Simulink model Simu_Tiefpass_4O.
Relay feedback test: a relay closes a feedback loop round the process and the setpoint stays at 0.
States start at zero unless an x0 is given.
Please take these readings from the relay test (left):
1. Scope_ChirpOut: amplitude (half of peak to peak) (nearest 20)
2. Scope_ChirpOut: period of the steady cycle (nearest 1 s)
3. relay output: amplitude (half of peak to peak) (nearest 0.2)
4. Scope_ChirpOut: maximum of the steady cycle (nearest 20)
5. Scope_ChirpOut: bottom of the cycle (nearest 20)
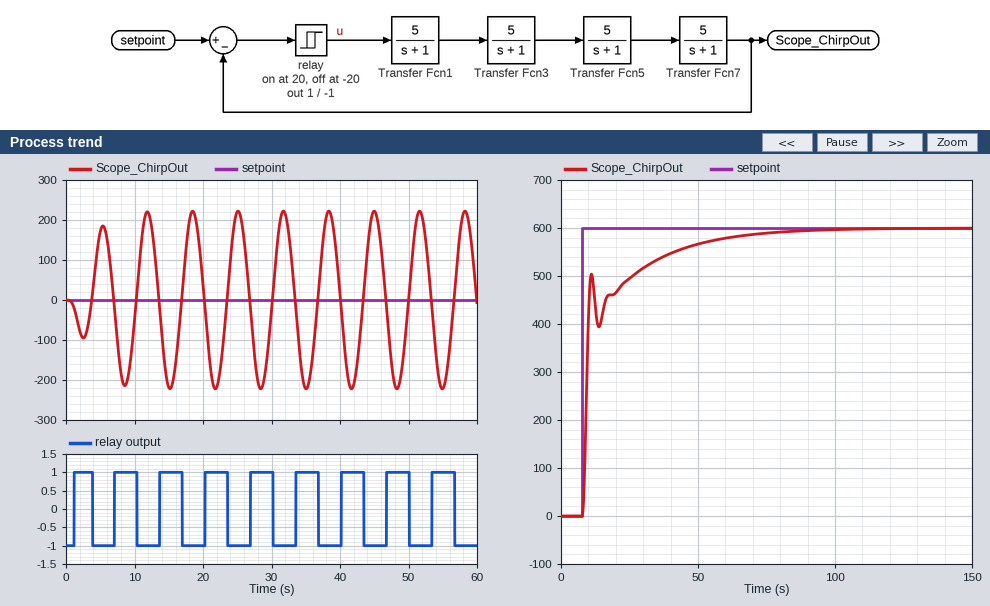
220
7 s
1.0
220
-220
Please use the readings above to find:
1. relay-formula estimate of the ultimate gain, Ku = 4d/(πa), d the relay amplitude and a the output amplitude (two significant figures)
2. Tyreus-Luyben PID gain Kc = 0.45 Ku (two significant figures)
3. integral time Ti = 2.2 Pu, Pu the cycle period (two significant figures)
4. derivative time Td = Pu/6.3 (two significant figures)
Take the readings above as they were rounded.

0.0058
0.0026
15 s
1.1 s
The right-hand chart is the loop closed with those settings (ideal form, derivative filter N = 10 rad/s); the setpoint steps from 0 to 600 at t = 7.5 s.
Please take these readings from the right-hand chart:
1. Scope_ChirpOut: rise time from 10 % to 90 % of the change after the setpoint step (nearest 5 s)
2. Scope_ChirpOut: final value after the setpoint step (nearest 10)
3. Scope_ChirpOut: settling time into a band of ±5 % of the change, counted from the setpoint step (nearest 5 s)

30 s
600
45 s
